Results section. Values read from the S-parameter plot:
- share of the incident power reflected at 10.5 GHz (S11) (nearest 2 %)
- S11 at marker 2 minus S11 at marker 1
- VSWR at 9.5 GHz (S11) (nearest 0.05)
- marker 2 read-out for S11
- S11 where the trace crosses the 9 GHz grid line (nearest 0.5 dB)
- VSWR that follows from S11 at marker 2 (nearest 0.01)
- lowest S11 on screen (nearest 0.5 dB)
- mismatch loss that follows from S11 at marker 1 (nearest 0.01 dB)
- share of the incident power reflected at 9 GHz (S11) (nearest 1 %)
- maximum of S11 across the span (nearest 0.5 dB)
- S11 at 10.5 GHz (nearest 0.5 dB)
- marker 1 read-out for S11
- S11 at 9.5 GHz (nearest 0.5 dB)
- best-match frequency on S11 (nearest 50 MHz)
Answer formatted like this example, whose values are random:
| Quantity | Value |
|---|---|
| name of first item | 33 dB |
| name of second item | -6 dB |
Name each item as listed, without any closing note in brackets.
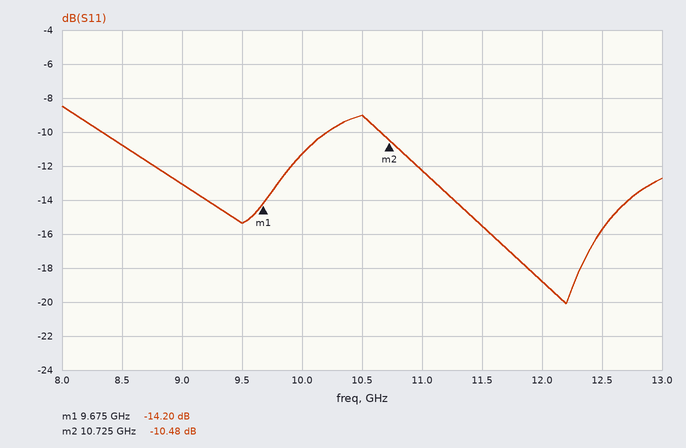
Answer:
| Quantity | Value |
|---|---|
| share of the incident power reflected at 10.5 GHz (S11) | 12 % |
| S11 at marker 2 minus S11 at marker 1 | 3.72 dB |
| VSWR at 9.5 GHz (S11) | 1.40 |
| marker 2 read-out for S11 | -10.48 dB |
| S11 where the trace crosses the 9 GHz grid line | -13.0 dB |
| VSWR that follows from S11 at marker 2 | 1.85 |
| lowest S11 on screen | -20.0 dB |
| mismatch loss that follows from S11 at marker 1 | 0.17 dB |
| share of the incident power reflected at 9 GHz (S11) | 5 % |
| maximum of S11 across the span | -8.5 dB |
| S11 at 10.5 GHz | -9.0 dB |
| marker 1 read-out for S11 | -14.20 dB |
| S11 at 9.5 GHz | -15.5 dB |
| best-match frequency on S11 | 12.20 GHz |
